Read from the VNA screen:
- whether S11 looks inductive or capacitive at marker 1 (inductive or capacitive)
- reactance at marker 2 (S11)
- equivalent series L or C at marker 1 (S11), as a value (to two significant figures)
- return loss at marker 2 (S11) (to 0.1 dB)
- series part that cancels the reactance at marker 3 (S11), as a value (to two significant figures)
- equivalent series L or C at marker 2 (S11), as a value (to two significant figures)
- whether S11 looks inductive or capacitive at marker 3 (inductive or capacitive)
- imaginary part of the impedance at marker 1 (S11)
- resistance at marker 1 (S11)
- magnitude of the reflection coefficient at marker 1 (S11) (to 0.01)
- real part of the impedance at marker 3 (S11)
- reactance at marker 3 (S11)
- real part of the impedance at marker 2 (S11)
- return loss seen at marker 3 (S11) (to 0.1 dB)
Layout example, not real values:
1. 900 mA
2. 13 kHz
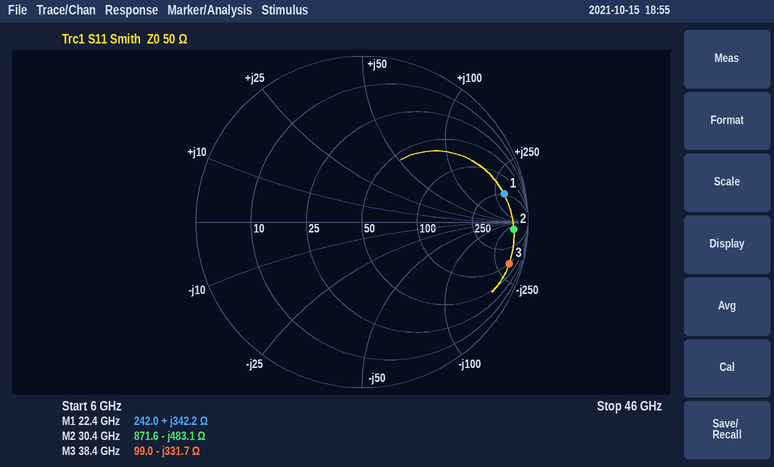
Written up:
1. inductive
2. -483.1 Ω
3. 2.4 nH
4. 0.8 dB
5. 1.4 nH
6. 11 fF
7. capacitive
8. +342.2 Ω
9. 242.0 Ω
10. 0.87
11. 99.0 Ω
12. -331.7 Ω
13. 871.6 Ω
14. 0.7 dB
